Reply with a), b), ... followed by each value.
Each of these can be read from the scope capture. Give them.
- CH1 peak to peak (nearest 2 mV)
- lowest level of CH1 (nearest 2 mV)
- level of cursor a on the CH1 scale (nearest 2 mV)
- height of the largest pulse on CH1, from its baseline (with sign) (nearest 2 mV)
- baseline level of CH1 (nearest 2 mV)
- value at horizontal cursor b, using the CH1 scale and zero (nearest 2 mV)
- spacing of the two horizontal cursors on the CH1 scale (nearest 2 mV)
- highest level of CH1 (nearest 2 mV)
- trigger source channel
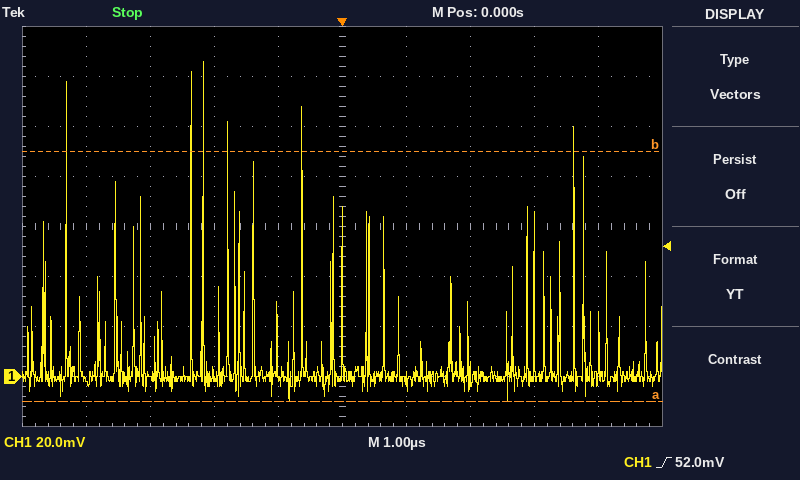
a) 136 mV
b) -10 mV
c) -10 mV
d) +126 mV
e) 0 mV
f) 90 mV
g) 100 mV
h) 126 mV
i) CH1
